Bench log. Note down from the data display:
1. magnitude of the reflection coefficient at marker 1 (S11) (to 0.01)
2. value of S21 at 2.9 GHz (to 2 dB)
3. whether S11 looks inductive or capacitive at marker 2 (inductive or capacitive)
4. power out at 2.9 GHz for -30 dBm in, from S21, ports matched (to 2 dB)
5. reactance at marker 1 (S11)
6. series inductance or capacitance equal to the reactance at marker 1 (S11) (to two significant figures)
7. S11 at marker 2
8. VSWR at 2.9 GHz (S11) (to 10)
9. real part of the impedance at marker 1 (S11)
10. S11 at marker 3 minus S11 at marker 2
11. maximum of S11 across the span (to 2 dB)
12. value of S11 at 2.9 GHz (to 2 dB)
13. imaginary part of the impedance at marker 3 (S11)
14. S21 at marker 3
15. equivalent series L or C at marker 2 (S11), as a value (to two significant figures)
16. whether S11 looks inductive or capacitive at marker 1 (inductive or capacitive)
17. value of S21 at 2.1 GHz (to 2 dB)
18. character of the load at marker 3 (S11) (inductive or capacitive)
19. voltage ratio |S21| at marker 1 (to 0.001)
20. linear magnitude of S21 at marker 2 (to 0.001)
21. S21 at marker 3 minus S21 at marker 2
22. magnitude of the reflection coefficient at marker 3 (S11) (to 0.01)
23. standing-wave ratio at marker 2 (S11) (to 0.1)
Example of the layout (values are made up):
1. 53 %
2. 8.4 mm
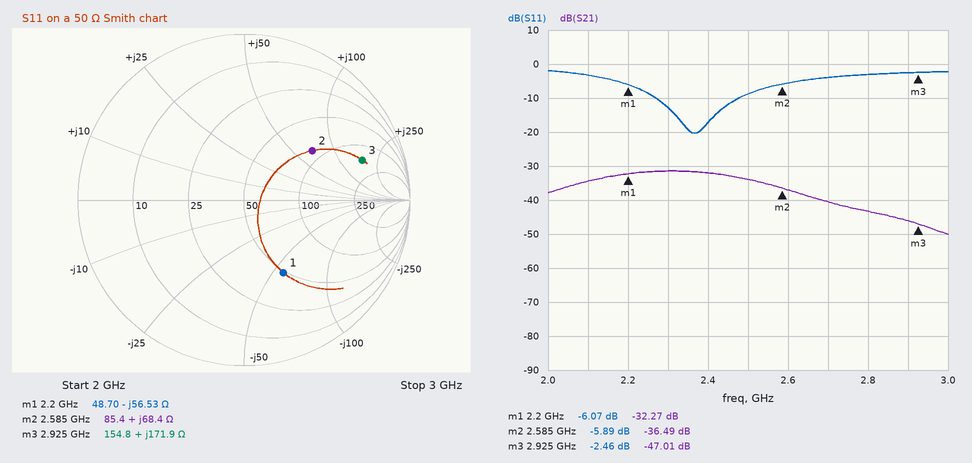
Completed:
1. 0.50
2. -46 dB
3. inductive
4. -76 dBm
5. -56.53 Ω
6. 1.3 pF
7. -5.89 dB
8. 10
9. 48.70 Ω
10. 3.43 dB
11. -2 dB
12. -2 dB
13. +171.9 Ω
14. -47.01 dB
15. 4.2 nH
16. capacitive
17. -34 dB
18. inductive
19. 0.024
20. 0.015
21. -10.52 dB
22. 0.75
23. 3.1
